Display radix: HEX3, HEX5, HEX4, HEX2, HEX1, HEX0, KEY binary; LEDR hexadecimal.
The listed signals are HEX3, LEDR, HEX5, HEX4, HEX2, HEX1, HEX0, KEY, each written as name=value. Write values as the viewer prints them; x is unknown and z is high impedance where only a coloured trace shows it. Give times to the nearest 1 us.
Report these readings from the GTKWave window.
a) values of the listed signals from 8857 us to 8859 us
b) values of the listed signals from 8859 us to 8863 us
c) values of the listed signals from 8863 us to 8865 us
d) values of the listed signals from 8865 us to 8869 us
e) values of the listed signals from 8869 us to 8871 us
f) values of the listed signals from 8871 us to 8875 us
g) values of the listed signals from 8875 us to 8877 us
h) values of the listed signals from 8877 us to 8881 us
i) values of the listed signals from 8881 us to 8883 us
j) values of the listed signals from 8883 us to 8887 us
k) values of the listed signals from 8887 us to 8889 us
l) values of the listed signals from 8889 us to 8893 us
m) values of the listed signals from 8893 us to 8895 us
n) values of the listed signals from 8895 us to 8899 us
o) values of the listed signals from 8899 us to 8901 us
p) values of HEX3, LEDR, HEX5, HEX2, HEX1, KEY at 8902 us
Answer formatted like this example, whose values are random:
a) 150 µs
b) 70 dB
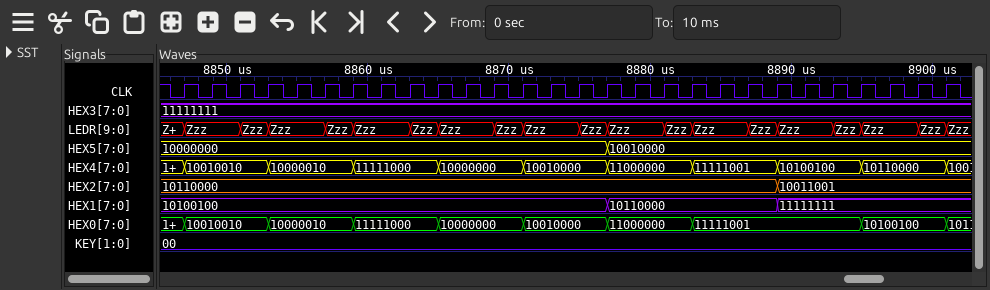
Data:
a) HEX3=11111111, LEDR=Zzz, HEX5=10000000, HEX4=10000010, HEX2=10110000, HEX1=10100100, HEX0=10000010, KEY=00
b) HEX3=11111111, LEDR=Zzz, HEX5=10000000, HEX4=11111000, HEX2=10110000, HEX1=10100100, HEX0=11111000, KEY=00
c) HEX3=11111111, LEDR=Zzz, HEX5=10000000, HEX4=11111000, HEX2=10110000, HEX1=10100100, HEX0=11111000, KEY=00
d) HEX3=11111111, LEDR=Zzz, HEX5=10000000, HEX4=10000000, HEX2=10110000, HEX1=10100100, HEX0=10000000, KEY=00
e) HEX3=11111111, LEDR=Zzz, HEX5=10000000, HEX4=10000000, HEX2=10110000, HEX1=10100100, HEX0=10000000, KEY=00
f) HEX3=11111111, LEDR=Zzz, HEX5=10000000, HEX4=10010000, HEX2=10110000, HEX1=10100100, HEX0=10010000, KEY=00
g) HEX3=11111111, LEDR=Zzz, HEX5=10000000, HEX4=10010000, HEX2=10110000, HEX1=10100100, HEX0=10010000, KEY=00
h) HEX3=11111111, LEDR=Zzz, HEX5=10010000, HEX4=11000000, HEX2=10110000, HEX1=10110000, HEX0=11000000, KEY=00
i) HEX3=11111111, LEDR=Zzz, HEX5=10010000, HEX4=11000000, HEX2=10110000, HEX1=10110000, HEX0=11000000, KEY=00
j) HEX3=11111111, LEDR=Zzz, HEX5=10010000, HEX4=11111001, HEX2=10110000, HEX1=10110000, HEX0=11111001, KEY=00
k) HEX3=11111111, LEDR=Zzz, HEX5=10010000, HEX4=11111001, HEX2=10110000, HEX1=10110000, HEX0=11111001, KEY=00
l) HEX3=11111111, LEDR=Zzz, HEX5=10010000, HEX4=10100100, HEX2=10011001, HEX1=11111111, HEX0=11111001, KEY=00
m) HEX3=11111111, LEDR=Zzz, HEX5=10010000, HEX4=10100100, HEX2=10011001, HEX1=11111111, HEX0=11111001, KEY=00
n) HEX3=11111111, LEDR=Zzz, HEX5=10010000, HEX4=10110000, HEX2=10011001, HEX1=11111111, HEX0=10100100, KEY=00
o) HEX3=11111111, LEDR=Zzz, HEX5=10010000, HEX4=10110000, HEX2=10011001, HEX1=11111111, HEX0=10100100, KEY=00
p) HEX3=11111111, LEDR=Zzz, HEX5=10010000, HEX2=10011001, HEX1=11111111, KEY=00
